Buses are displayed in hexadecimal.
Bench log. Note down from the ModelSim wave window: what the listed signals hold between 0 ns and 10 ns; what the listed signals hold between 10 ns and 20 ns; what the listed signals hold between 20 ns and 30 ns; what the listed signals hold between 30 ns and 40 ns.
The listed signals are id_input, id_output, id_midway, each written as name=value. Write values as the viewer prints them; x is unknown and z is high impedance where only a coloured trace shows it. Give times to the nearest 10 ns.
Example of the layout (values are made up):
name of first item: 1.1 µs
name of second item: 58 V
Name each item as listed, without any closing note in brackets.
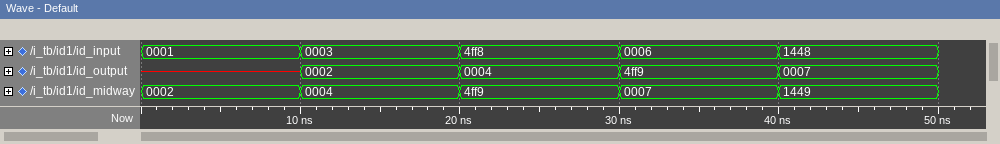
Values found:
what the listed signals hold between 0 ns and 10 ns: id_input=0001, id_output=x, id_midway=0002
what the listed signals hold between 10 ns and 20 ns: id_input=0003, id_output=0002, id_midway=0004
what the listed signals hold between 20 ns and 30 ns: id_input=4ff8, id_output=0004, id_midway=4ff9
what the listed signals hold between 30 ns and 40 ns: id_input=0006, id_output=4ff9, id_midway=0007
